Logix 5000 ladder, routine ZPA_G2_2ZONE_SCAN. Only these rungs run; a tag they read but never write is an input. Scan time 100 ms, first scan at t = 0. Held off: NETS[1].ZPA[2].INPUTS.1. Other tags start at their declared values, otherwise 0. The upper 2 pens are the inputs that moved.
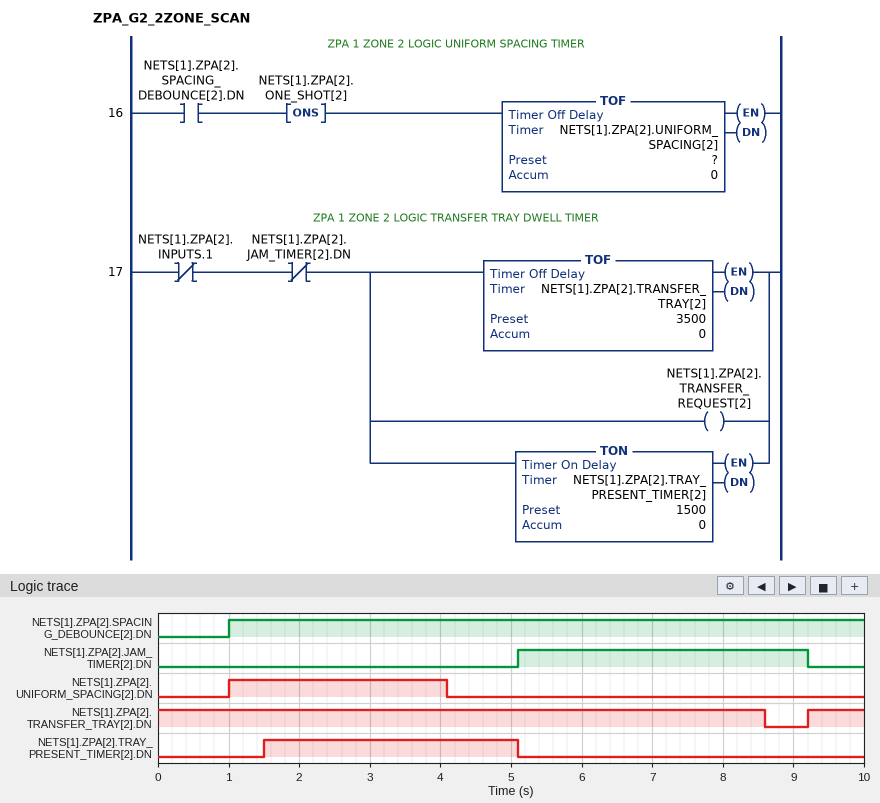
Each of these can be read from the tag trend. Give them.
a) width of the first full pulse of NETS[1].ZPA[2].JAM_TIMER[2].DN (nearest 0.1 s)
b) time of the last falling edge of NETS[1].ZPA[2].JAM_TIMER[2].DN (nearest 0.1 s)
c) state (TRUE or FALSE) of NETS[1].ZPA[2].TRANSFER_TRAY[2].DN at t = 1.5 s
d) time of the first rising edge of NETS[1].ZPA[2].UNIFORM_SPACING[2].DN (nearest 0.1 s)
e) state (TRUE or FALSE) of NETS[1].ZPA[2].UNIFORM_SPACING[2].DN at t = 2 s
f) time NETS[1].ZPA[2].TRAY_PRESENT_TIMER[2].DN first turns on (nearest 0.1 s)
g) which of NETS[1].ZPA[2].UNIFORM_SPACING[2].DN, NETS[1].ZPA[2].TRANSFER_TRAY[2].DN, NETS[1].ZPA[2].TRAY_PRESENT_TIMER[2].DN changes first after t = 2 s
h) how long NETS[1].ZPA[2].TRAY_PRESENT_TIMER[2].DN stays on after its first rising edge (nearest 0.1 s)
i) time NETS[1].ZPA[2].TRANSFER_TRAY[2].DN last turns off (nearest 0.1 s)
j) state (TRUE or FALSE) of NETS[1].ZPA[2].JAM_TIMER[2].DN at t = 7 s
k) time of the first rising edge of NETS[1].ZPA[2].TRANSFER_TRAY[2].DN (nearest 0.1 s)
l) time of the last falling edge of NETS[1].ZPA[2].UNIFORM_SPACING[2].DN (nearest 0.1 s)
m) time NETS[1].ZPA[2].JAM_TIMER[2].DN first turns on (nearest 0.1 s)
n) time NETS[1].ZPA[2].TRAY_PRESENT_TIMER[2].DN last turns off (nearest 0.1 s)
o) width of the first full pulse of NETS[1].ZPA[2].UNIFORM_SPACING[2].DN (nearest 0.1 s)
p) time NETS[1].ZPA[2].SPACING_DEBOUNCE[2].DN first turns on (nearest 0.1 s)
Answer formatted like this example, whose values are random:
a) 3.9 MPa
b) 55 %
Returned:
a) 4.1 s
b) 9.2 s
c) TRUE
d) 1.0 s
e) TRUE
f) 1.5 s
g) NETS[1].ZPA[2].UNIFORM_SPACING[2].DN
h) 3.6 s
i) 8.6 s
j) TRUE
k) 9.2 s
l) 4.1 s
m) 5.1 s
n) 5.1 s
o) 3.1 s
p) 1.0 s
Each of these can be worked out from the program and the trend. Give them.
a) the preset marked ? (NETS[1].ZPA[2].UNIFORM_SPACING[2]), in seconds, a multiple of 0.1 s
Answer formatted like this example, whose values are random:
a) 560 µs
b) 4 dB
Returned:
a) 3.0 s
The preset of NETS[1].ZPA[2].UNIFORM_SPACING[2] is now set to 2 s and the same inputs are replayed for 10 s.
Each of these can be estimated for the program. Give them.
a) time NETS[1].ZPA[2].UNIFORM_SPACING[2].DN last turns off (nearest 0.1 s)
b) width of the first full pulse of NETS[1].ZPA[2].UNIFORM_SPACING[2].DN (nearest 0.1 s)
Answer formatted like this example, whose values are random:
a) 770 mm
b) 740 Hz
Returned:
a) 3.1 s
b) 2.1 s
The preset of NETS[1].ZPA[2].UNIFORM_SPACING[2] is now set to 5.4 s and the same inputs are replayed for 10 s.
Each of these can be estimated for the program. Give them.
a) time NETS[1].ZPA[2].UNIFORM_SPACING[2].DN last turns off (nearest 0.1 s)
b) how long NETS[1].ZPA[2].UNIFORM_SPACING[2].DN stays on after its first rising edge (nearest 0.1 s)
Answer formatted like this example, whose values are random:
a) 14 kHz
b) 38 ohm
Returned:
a) 6.5 s
b) 5.5 s
